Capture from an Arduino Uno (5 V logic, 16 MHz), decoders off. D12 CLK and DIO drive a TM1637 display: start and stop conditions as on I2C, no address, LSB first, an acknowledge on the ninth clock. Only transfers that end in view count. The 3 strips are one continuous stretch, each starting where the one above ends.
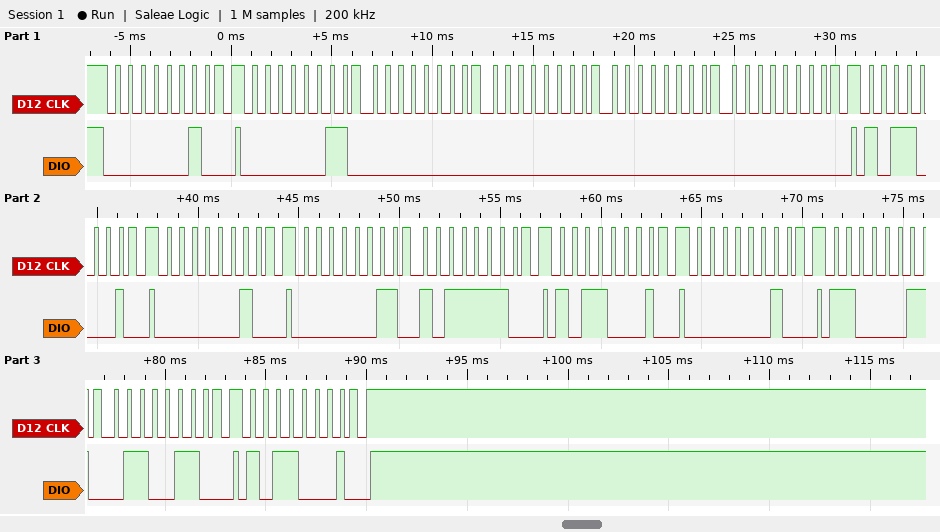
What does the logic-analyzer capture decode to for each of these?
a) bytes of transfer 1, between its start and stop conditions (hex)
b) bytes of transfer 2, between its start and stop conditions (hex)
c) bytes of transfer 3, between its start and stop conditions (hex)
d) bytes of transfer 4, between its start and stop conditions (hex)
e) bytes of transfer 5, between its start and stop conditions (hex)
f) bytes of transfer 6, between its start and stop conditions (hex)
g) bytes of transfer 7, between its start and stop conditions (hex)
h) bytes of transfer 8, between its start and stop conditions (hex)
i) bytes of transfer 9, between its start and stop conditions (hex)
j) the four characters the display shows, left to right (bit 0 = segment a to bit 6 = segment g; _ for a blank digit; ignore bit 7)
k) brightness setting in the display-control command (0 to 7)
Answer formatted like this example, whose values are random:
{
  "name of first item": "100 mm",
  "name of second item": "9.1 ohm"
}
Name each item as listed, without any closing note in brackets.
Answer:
{
  "bytes of transfer 1, between its start and stop conditions": "40",
  "bytes of transfer 2, between its start and stop conditions": "C0 00 00 00 00",
  "bytes of transfer 3, between its start and stop conditions": "8D",
  "bytes of transfer 4, between its start and stop conditions": "40",
  "bytes of transfer 5, between its start and stop conditions": "C0 7D",
  "bytes of transfer 6, between its start and stop conditions": "8D",
  "bytes of transfer 7, between its start and stop conditions": "40",
  "bytes of transfer 8, between its start and stop conditions": "C3 66",
  "bytes of transfer 9, between its start and stop conditions": "8D",
  "the four characters the display shows, left to right": "6__4",
  "brightness setting in the display-control command": "5"
}
